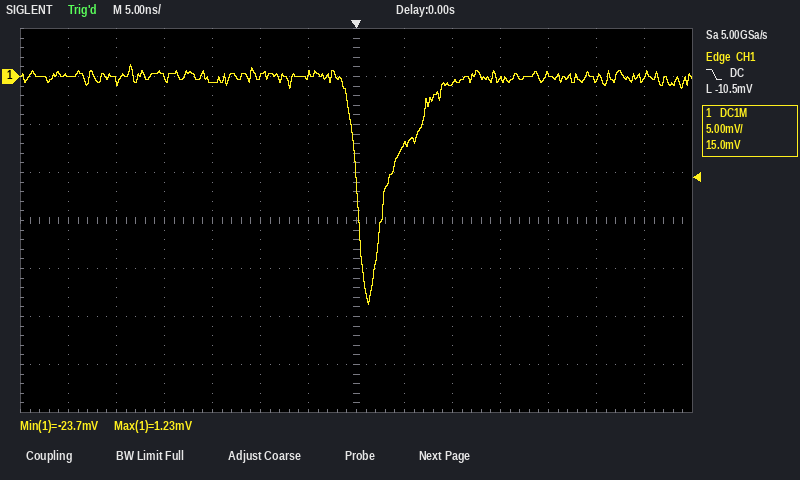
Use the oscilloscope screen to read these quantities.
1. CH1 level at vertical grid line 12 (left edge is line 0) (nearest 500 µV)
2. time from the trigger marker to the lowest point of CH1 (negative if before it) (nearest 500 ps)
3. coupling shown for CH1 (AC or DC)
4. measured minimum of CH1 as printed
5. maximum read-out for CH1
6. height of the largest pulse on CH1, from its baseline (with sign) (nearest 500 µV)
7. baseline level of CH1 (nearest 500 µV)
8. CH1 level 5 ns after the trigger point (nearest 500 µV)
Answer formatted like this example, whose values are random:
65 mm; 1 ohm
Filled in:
-500 µV; +1.5 ns; DC; -23.7 mV; 1.23 mV; -23.5 mV; 0.0 mV; -7.0 mV
